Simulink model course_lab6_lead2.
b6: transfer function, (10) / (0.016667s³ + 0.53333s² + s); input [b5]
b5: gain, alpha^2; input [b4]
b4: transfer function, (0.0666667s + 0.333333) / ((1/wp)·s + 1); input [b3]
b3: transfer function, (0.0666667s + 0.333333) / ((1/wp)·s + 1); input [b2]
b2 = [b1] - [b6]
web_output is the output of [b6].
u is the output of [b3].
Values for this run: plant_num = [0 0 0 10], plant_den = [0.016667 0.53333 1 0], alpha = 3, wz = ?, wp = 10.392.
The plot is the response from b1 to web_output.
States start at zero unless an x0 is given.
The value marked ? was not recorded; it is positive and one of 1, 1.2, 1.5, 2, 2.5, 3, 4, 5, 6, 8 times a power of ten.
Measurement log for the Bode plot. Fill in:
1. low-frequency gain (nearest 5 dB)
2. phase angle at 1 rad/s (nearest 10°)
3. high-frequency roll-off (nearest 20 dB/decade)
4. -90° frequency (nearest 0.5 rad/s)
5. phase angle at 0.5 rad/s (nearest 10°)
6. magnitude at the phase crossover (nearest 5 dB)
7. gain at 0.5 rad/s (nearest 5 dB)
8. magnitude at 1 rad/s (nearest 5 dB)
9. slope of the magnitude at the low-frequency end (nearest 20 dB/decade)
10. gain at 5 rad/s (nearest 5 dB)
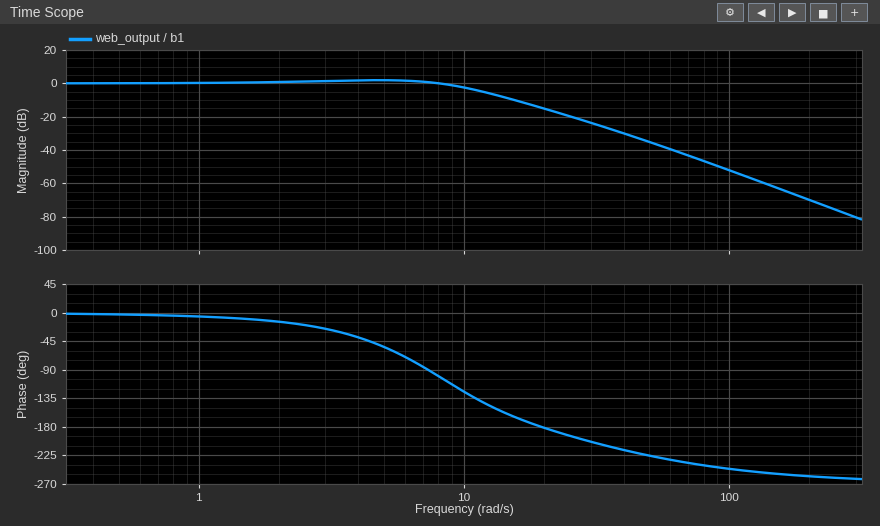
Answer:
0 dB
-10°
-60 dB/decade
7.5 rad/s
0°
-15 dB
0 dB
0 dB
0 dB/decade
0 dB
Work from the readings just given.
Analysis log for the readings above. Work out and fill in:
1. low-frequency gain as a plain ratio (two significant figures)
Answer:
1.0
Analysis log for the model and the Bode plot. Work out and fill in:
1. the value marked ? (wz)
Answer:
5
